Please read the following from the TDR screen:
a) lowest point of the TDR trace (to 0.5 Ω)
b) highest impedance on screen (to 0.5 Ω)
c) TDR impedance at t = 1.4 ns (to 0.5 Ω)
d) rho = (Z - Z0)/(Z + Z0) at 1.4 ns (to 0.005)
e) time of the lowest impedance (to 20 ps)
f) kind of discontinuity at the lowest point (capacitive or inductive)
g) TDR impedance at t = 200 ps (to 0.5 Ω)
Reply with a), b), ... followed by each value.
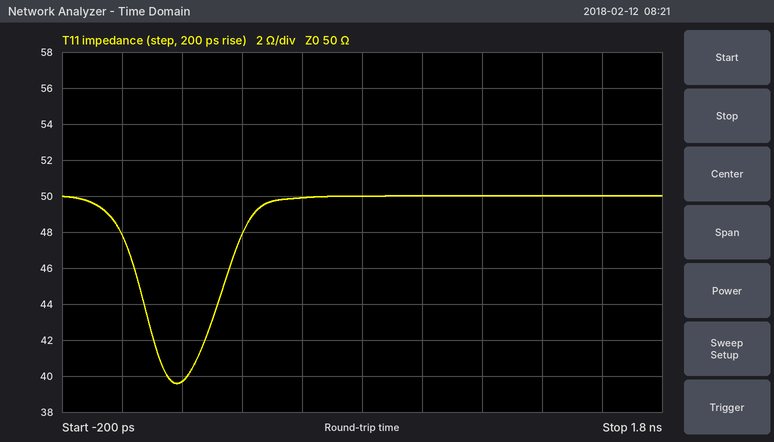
a) 39.5 Ω
b) 50.0 Ω
c) 50.0 Ω
d) 0.000
e) 180 ps
f) capacitive
g) 39.5 Ω
